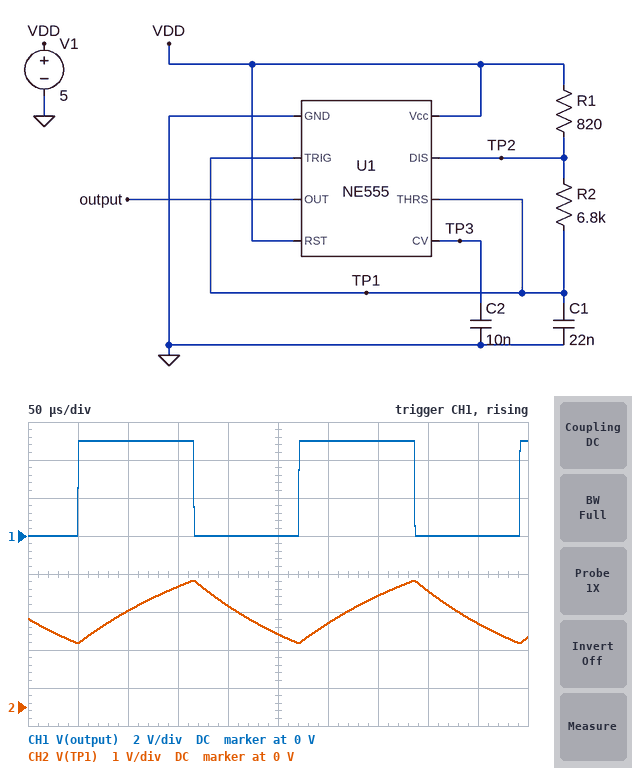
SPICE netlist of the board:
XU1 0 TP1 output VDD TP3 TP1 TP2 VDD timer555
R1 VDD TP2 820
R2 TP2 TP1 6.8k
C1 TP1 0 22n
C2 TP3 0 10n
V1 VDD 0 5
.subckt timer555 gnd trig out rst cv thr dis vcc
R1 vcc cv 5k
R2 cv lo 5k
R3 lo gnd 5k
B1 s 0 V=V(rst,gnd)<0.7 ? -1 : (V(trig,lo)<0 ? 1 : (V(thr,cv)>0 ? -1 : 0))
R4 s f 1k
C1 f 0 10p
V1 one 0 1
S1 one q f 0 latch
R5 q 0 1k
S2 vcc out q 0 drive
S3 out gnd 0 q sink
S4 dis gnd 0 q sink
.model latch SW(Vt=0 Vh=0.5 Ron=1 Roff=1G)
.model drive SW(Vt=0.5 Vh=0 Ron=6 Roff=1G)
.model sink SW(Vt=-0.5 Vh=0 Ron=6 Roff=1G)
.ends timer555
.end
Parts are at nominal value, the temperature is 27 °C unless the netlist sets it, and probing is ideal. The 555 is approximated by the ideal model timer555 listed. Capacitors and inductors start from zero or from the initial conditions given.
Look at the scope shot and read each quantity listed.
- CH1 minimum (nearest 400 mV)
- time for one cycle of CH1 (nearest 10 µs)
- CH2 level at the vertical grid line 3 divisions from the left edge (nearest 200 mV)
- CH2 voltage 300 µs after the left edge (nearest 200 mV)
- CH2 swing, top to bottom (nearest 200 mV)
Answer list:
0 V
220 µs
3.2 V
2.2 V
1.6 V
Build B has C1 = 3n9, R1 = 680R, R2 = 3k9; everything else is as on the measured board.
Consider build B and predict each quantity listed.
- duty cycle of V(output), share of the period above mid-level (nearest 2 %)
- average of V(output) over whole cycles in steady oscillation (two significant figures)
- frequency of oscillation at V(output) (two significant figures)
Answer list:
54 %
2.7 V
43 kHz
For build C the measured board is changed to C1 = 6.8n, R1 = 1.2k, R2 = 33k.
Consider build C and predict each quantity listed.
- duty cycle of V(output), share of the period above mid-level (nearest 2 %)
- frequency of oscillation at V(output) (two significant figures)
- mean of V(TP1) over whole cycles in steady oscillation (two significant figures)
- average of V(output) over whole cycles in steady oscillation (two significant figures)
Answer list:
50 %
3.1 kHz
2.5 V
2.5 V
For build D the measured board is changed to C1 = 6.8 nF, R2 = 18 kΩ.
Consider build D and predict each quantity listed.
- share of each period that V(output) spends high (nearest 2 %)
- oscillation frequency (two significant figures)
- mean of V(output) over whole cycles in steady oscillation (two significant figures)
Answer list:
50 %
5.7 kHz
2.5 V
